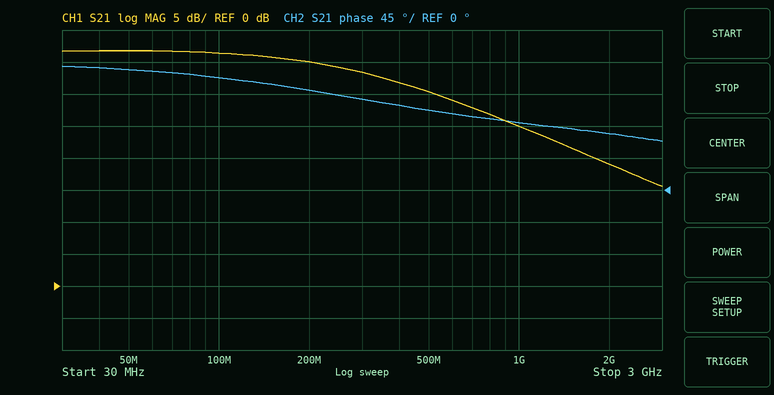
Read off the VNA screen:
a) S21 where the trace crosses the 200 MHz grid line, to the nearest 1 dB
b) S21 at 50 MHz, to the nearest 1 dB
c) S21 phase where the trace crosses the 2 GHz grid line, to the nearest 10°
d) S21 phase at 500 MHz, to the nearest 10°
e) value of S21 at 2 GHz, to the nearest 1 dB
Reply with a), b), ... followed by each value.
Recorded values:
a) 35 dB
b) 37 dB
c) 80°
d) 110°
e) 19 dB
